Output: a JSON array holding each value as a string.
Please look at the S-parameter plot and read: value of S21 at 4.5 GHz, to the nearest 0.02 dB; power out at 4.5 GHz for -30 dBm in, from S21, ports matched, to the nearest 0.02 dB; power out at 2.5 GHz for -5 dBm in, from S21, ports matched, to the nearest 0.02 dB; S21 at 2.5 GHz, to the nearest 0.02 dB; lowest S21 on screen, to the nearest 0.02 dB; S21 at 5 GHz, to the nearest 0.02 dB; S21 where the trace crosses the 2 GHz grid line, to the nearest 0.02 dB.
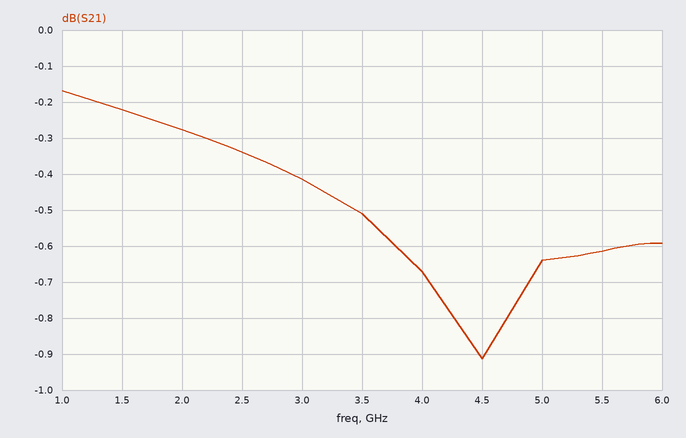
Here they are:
["-0.92 dB", "-30.92 dBm", "-5.34 dBm", "-0.34 dB", "-0.92 dB", "-0.64 dB", "-0.28 dB"]
